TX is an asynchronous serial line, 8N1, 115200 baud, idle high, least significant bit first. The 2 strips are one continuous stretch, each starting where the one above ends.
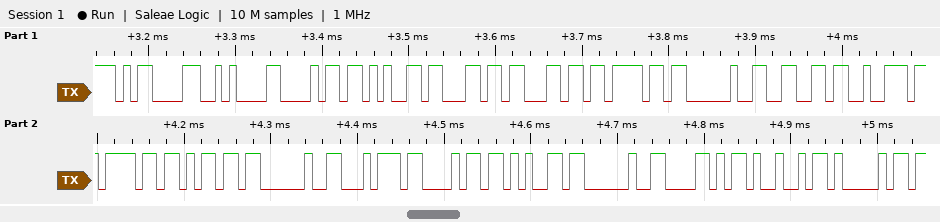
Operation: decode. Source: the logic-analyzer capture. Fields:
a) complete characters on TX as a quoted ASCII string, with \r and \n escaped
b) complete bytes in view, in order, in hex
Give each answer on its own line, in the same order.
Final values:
"\r\nhello from the XIA"
0D 0A 68 65 6C 6C 6F 20 66 72 6F 6D 20 74 68 65 20 58 49 41
